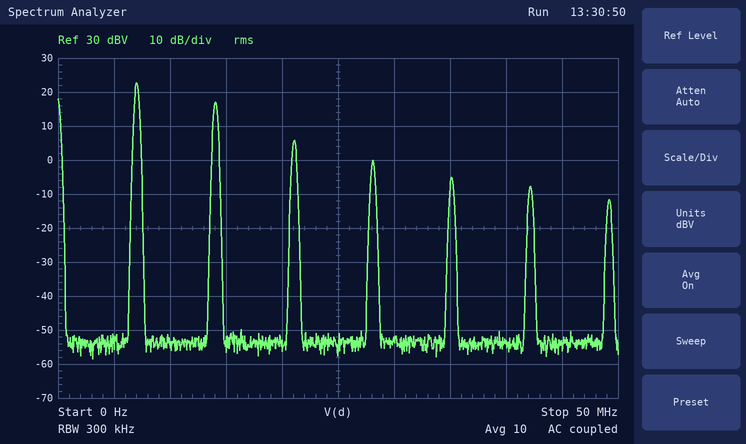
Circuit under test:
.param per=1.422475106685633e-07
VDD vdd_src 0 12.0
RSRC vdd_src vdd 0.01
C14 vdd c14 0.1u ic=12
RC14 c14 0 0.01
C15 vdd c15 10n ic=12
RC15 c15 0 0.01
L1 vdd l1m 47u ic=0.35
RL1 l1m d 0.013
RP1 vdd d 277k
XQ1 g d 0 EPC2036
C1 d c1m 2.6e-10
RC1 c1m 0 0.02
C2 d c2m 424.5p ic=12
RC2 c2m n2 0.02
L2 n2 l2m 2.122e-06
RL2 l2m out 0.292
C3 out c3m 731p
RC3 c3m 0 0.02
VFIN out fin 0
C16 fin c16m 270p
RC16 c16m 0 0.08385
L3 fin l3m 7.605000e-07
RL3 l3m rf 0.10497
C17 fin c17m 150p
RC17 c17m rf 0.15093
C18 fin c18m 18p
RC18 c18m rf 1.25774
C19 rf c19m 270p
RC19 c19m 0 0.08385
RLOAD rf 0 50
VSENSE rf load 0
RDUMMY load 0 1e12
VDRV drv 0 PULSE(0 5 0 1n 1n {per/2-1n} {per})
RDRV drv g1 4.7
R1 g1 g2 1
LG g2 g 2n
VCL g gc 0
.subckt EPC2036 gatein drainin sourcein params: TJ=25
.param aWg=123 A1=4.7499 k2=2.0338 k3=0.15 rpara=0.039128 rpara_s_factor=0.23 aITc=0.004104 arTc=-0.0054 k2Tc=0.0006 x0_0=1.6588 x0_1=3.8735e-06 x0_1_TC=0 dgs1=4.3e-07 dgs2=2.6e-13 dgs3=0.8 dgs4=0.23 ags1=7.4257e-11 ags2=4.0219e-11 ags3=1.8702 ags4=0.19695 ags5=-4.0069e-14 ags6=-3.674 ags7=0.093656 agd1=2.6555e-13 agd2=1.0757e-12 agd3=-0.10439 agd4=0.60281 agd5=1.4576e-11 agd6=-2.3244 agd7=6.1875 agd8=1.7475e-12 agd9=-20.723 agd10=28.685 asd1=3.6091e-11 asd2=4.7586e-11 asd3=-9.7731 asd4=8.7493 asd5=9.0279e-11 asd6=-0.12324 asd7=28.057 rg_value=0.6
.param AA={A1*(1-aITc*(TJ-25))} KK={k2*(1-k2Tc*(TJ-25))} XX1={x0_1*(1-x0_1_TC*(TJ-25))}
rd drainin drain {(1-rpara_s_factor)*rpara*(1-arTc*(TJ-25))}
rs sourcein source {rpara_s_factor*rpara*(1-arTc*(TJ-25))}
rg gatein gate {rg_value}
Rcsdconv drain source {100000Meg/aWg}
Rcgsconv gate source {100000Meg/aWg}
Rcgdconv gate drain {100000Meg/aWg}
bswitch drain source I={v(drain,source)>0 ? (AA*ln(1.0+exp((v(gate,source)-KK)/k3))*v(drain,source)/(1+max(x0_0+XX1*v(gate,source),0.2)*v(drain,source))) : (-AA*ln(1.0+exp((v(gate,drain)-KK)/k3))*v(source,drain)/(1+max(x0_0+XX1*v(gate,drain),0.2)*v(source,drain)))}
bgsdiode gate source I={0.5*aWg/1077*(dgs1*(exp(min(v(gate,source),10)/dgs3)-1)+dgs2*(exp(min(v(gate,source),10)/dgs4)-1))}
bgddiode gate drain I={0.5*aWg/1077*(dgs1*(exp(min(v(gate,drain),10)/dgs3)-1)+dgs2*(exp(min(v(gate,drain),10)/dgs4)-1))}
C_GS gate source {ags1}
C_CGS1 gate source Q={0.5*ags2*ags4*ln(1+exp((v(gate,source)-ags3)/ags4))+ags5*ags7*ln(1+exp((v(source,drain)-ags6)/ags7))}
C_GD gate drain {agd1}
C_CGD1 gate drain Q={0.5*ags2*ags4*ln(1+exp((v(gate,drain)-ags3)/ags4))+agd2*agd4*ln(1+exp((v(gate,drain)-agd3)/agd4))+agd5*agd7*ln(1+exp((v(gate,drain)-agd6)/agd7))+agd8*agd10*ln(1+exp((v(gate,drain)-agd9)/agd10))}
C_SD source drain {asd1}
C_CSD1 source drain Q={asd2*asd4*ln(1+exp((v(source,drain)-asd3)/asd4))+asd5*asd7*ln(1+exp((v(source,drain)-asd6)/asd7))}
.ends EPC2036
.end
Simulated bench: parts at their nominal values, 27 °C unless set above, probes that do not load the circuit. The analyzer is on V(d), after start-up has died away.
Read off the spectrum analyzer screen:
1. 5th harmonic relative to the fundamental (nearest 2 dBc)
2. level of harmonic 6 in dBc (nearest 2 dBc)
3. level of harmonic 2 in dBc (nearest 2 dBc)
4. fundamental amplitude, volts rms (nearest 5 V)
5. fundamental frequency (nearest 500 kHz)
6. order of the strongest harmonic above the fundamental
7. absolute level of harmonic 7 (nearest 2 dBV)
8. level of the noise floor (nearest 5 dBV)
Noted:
-28 dBc
-30 dBc
-6 dBc
15 V
7.0 MHz
2
-12 dBV
-55 dBV
